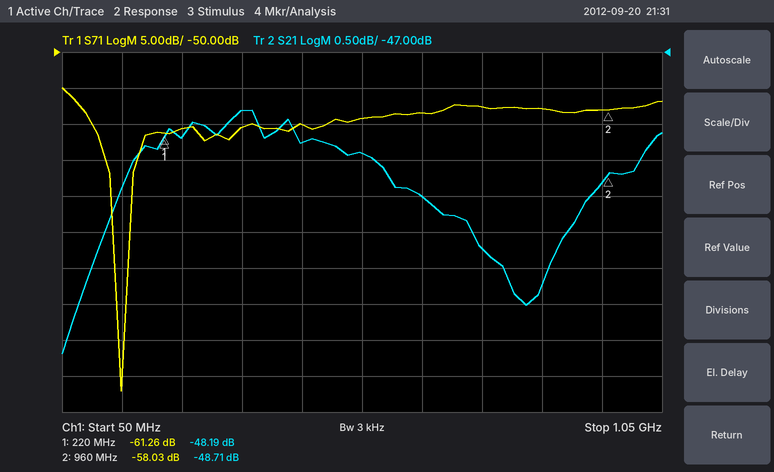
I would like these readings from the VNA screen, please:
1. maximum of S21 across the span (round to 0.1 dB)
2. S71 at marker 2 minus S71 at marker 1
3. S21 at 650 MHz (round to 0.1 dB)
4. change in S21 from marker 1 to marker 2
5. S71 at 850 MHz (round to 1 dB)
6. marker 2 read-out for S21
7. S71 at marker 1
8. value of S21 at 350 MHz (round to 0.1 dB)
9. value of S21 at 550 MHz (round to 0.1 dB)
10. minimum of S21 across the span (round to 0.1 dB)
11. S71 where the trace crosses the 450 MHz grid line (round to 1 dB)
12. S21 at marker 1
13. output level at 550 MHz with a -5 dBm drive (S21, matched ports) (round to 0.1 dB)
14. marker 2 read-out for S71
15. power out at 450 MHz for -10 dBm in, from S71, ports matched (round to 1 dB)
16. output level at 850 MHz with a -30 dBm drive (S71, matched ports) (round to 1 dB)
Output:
-47.8 dB
3.23 dB
-49.0 dB
-0.52 dB
-58 dB
-48.71 dB
-61.26 dB
-47.8 dB
-48.4 dB
-51.2 dB
-60 dB
-48.19 dB
-53.4 dBm
-58.03 dB
-70 dBm
-88 dBm
